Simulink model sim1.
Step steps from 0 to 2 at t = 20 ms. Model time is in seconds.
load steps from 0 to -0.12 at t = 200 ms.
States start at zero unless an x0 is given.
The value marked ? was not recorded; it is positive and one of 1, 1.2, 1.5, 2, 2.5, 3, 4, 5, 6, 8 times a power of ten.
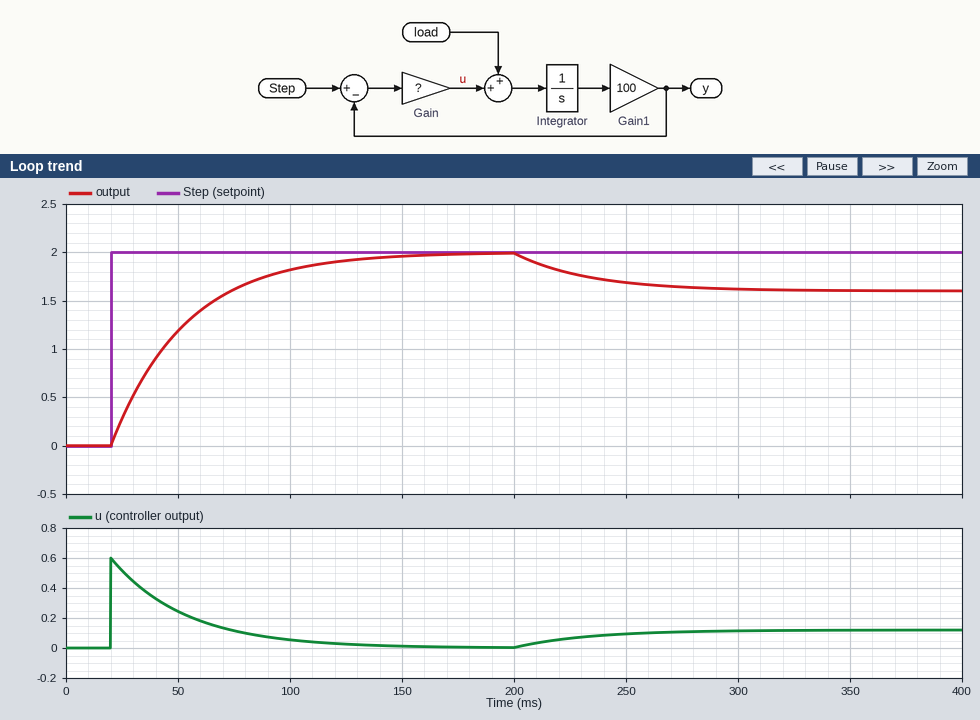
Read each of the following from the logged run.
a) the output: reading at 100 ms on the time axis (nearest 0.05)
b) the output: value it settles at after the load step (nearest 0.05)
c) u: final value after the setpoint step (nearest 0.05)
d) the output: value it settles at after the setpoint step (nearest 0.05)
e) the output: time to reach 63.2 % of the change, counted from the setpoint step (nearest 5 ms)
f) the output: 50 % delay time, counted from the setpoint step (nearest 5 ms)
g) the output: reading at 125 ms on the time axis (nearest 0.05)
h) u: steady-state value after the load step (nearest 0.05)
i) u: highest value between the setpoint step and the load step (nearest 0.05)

1.80
1.60
0.00
2.00
35 ms
25 ms
1.90
0.10
0.60
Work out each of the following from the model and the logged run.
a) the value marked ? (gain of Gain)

0.3
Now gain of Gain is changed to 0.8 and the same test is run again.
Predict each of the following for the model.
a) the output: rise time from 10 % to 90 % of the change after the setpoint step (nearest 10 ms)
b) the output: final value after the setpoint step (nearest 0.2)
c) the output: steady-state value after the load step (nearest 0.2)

30 ms
2.0
1.8
